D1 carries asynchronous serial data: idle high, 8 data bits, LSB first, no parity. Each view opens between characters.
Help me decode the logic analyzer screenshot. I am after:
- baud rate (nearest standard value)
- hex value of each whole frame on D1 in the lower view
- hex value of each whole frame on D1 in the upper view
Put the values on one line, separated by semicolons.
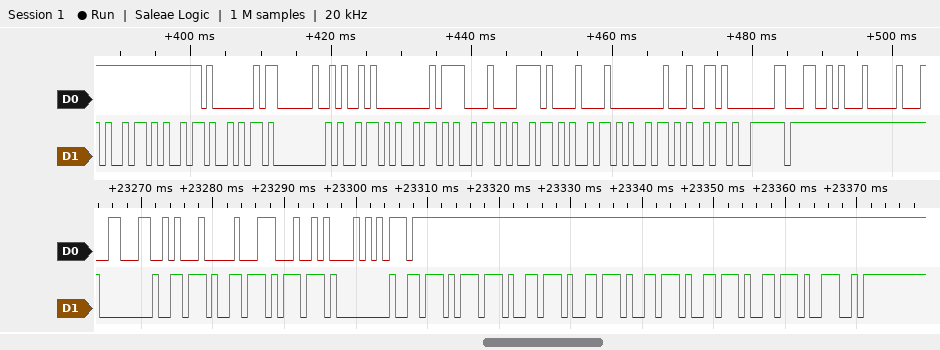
1200 baud; 00, 76, 76, 77, 00, 76, 77, 76, 76, 76, 76, 76, 4E; 69, 69, 6A, 00, 69, 69, 69, 69, 69, 69, 69, 7E
